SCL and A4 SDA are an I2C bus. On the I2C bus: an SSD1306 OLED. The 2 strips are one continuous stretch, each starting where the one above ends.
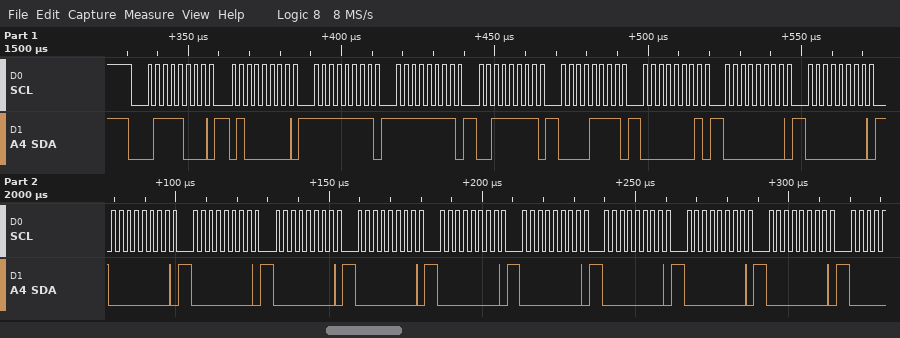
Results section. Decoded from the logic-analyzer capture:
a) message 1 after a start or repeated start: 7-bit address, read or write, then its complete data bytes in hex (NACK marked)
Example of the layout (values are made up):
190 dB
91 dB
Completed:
0x3C write: 40 FF FF 3F 0F 01 00 00 00 00 00 00 00 00 00 00 00
